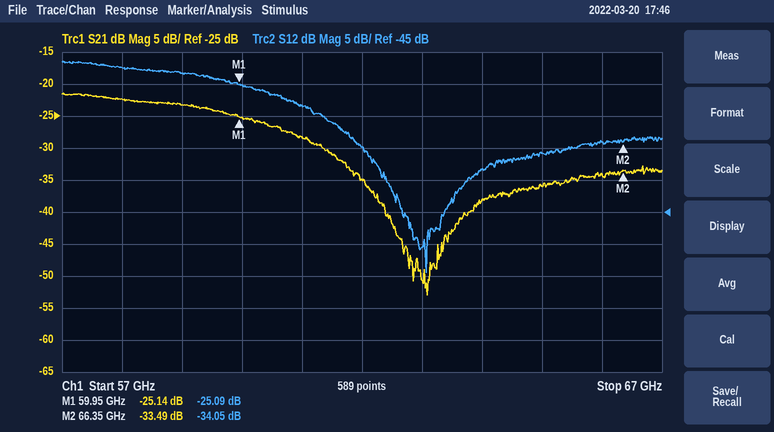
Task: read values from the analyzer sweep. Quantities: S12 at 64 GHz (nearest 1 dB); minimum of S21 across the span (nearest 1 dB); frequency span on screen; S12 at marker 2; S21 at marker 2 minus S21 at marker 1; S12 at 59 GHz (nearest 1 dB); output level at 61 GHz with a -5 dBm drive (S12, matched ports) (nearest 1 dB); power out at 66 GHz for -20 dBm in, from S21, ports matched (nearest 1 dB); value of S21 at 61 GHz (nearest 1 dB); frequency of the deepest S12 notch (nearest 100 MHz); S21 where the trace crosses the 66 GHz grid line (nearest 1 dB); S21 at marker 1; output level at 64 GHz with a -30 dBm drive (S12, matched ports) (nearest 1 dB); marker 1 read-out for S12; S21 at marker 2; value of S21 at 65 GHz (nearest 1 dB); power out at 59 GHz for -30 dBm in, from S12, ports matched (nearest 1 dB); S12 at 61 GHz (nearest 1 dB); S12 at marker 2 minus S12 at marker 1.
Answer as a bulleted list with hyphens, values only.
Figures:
- -38 dB
- -53 dB
- 10 GHz
- -34.05 dB
- -8.35 dB
- -23 dB
- -33 dBm
- -54 dBm
- -28 dB
- 63.1 GHz
- -34 dB
- -25.14 dB
- -68 dBm
- -25.09 dB
- -33.49 dB
- -36 dB
- -53 dBm
- -28 dB
- -8.96 dB
